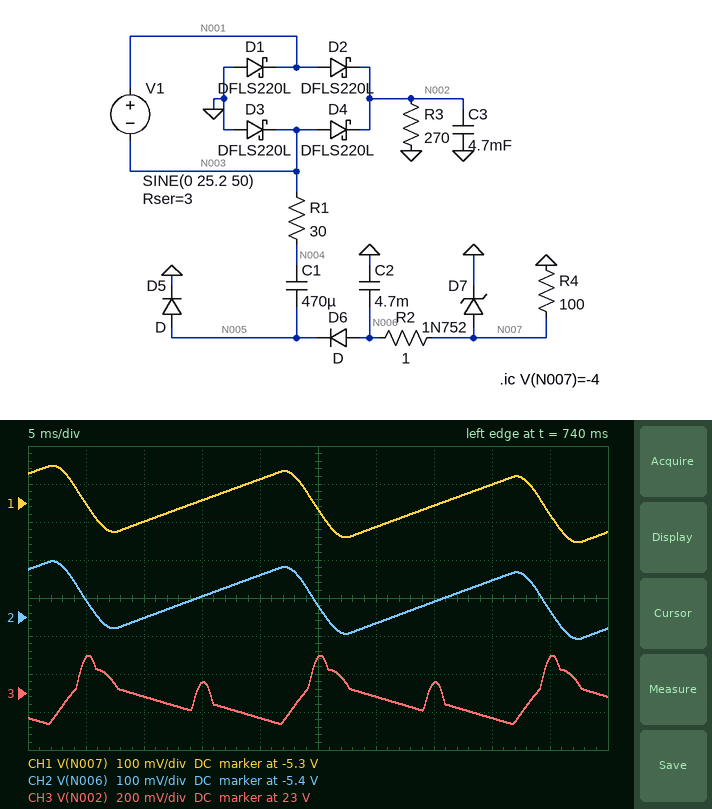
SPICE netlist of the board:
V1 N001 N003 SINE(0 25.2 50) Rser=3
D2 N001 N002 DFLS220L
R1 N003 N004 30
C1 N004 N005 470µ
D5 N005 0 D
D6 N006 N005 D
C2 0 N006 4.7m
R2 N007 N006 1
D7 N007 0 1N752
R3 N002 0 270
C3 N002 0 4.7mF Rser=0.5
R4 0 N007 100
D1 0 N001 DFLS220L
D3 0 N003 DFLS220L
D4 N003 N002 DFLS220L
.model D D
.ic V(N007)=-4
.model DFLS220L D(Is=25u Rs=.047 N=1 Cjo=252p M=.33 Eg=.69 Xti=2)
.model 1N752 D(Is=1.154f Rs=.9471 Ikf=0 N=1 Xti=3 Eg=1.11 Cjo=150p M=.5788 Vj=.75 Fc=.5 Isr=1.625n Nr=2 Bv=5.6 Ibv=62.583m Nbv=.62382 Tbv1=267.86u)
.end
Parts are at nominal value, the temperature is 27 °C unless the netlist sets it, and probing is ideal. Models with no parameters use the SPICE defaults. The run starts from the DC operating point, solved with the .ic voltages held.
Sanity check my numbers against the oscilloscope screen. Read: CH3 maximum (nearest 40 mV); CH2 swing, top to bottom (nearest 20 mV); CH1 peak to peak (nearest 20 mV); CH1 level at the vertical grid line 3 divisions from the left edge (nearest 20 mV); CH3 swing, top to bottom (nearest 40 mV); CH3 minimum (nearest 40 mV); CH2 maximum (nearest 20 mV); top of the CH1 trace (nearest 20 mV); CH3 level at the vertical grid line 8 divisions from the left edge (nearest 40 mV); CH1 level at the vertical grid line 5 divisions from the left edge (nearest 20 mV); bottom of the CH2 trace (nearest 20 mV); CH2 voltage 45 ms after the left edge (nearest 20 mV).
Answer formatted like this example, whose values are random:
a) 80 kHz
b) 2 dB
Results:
a) 23.20 V
b) 200 mV
c) 200 mV
d) -5.30 V
e) 360 mV
f) 22.84 V
g) -5.26 V
h) -5.20 V
i) 22.88 V
j) -5.32 V
k) -5.46 V
l) -5.38 V
